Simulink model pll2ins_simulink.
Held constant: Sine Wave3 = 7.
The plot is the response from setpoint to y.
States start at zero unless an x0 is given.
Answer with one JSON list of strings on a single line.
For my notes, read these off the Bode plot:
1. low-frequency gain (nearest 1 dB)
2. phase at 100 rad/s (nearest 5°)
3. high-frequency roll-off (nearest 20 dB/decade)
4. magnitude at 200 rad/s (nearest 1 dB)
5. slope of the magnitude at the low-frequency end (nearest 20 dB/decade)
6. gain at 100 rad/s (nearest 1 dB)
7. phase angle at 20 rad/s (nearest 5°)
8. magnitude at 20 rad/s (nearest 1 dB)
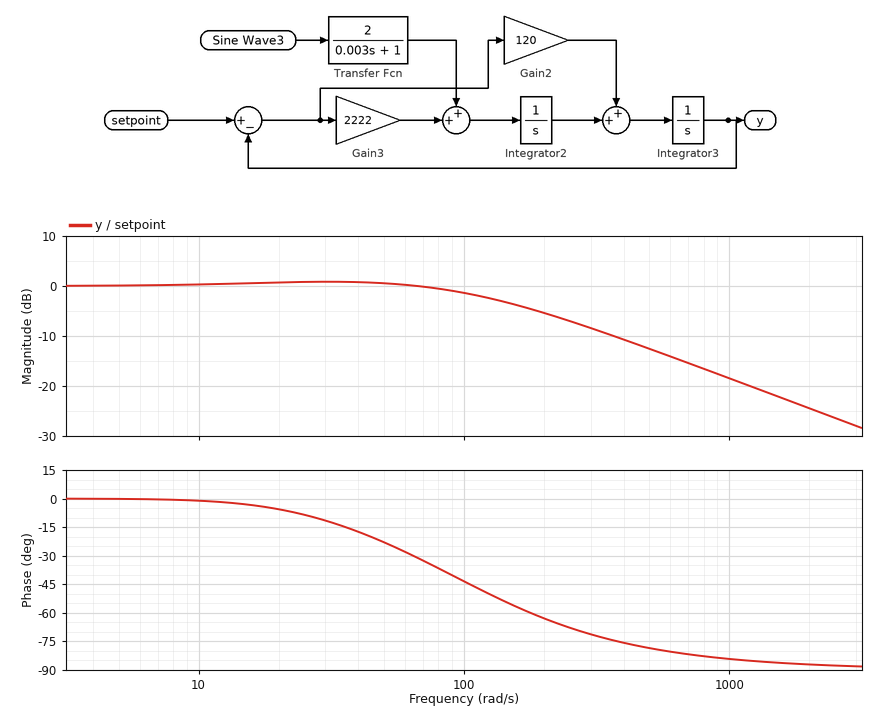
["0 dB", "-45°", "-20 dB/decade", "-5 dB", "0 dB/decade", "-1 dB", "-5°", "1 dB"]
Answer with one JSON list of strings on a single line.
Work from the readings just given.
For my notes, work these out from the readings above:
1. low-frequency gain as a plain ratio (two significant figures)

["1.0"]
